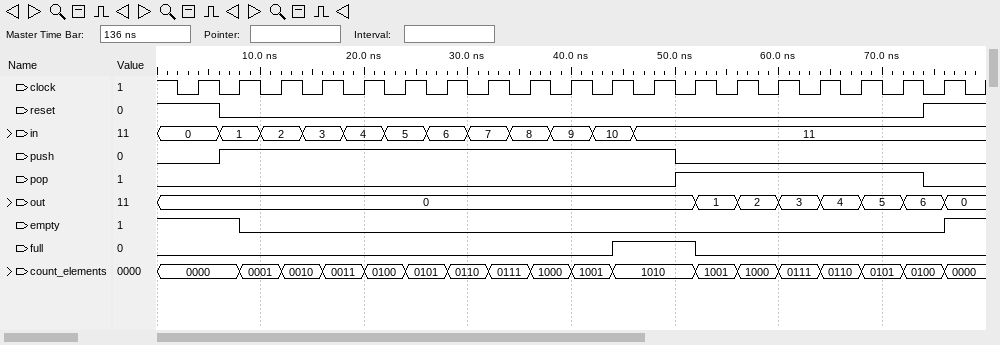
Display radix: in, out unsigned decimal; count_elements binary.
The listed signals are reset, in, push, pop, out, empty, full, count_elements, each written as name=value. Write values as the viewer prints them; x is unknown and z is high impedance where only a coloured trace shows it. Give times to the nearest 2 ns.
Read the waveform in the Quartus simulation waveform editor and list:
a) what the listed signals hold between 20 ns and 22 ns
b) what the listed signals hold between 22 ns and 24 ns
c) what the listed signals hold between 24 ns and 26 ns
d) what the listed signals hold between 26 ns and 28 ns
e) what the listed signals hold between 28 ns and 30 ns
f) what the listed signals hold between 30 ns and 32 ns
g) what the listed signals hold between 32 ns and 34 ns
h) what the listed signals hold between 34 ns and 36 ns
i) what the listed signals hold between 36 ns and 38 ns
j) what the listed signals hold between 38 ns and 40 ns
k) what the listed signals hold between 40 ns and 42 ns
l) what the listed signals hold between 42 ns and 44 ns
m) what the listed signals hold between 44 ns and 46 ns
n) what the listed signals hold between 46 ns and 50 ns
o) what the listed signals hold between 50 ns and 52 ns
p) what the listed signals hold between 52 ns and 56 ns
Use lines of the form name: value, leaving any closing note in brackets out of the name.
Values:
what the listed signals hold between 20 ns and 22 ns: reset=0, in=4, push=1, pop=0, out=0, empty=0, full=0, count_elements=0100
what the listed signals hold between 22 ns and 24 ns: reset=0, in=5, push=1, pop=0, out=0, empty=0, full=0, count_elements=0100
what the listed signals hold between 24 ns and 26 ns: reset=0, in=5, push=1, pop=0, out=0, empty=0, full=0, count_elements=0101
what the listed signals hold between 26 ns and 28 ns: reset=0, in=6, push=1, pop=0, out=0, empty=0, full=0, count_elements=0101
what the listed signals hold between 28 ns and 30 ns: reset=0, in=6, push=1, pop=0, out=0, empty=0, full=0, count_elements=0110
what the listed signals hold between 30 ns and 32 ns: reset=0, in=7, push=1, pop=0, out=0, empty=0, full=0, count_elements=0110
what the listed signals hold between 32 ns and 34 ns: reset=0, in=7, push=1, pop=0, out=0, empty=0, full=0, count_elements=0111
what the listed signals hold between 34 ns and 36 ns: reset=0, in=8, push=1, pop=0, out=0, empty=0, full=0, count_elements=0111
what the listed signals hold between 36 ns and 38 ns: reset=0, in=8, push=1, pop=0, out=0, empty=0, full=0, count_elements=1000
what the listed signals hold between 38 ns and 40 ns: reset=0, in=9, push=1, pop=0, out=0, empty=0, full=0, count_elements=1000
what the listed signals hold between 40 ns and 42 ns: reset=0, in=9, push=1, pop=0, out=0, empty=0, full=0, count_elements=1001
what the listed signals hold between 42 ns and 44 ns: reset=0, in=10, push=1, pop=0, out=0, empty=0, full=0, count_elements=1001
what the listed signals hold between 44 ns and 46 ns: reset=0, in=10, push=1, pop=0, out=0, empty=0, full=1, count_elements=1010
what the listed signals hold between 46 ns and 50 ns: reset=0, in=11, push=1, pop=0, out=0, empty=0, full=1, count_elements=1010
what the listed signals hold between 50 ns and 52 ns: reset=0, in=11, push=0, pop=1, out=0, empty=0, full=1, count_elements=1010
what the listed signals hold between 52 ns and 56 ns: reset=0, in=11, push=0, pop=1, out=1, empty=0, full=0, count_elements=1001
